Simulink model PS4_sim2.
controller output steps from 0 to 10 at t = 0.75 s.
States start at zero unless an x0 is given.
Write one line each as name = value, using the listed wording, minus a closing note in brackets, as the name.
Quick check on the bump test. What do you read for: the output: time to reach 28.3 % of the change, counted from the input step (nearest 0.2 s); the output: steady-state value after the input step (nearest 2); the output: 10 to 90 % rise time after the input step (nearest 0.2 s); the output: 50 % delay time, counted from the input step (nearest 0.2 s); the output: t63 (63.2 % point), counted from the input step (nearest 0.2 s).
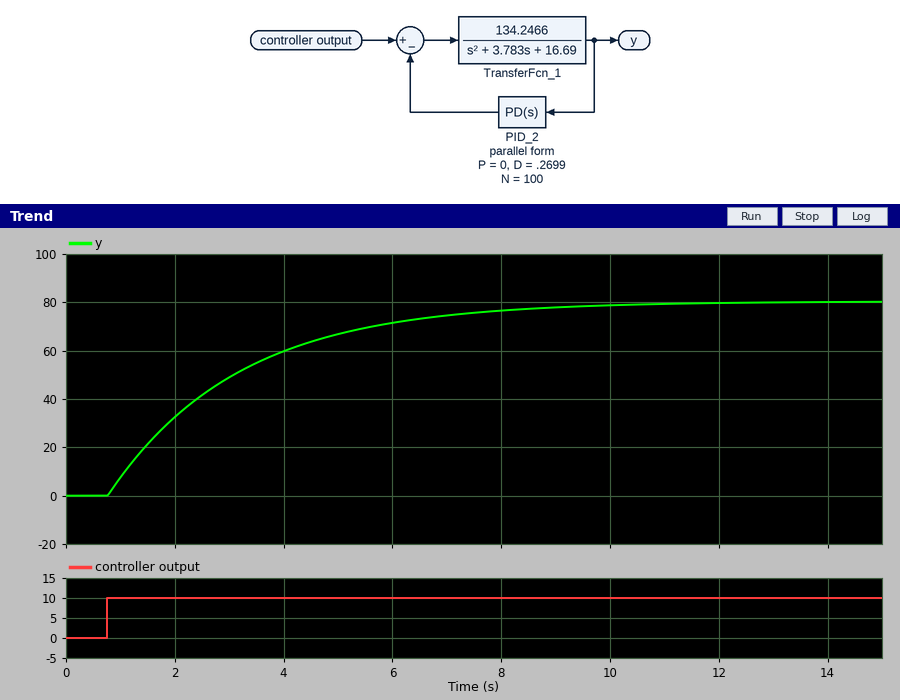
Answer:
the output: time to reach 28.3 % of the change, counted from the input step = 0.8 s
the output: steady-state value after the input step = 80
the output: 10 to 90 % rise time after the input step = 5.2 s
the output: 50 % delay time, counted from the input step = 1.6 s
the output: t63 (63.2 % point), counted from the input step = 2.4 s
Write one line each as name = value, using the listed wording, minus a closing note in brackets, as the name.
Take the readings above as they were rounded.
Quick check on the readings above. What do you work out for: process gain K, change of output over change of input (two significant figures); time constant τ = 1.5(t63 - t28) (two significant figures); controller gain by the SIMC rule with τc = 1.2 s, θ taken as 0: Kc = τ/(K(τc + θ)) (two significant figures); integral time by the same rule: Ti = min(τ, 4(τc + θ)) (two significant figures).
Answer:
process gain K, change of output over change of input = 8.0
time constant τ = 1.5(t63 - t28) = 2.4 s
controller gain by the SIMC rule with τc = 1.2 s, θ taken as 0: Kc = τ/(K(τc + θ)) = 0.25
integral time by the same rule: Ti = min(τ, 4(τc + θ)) = 2.4 s
